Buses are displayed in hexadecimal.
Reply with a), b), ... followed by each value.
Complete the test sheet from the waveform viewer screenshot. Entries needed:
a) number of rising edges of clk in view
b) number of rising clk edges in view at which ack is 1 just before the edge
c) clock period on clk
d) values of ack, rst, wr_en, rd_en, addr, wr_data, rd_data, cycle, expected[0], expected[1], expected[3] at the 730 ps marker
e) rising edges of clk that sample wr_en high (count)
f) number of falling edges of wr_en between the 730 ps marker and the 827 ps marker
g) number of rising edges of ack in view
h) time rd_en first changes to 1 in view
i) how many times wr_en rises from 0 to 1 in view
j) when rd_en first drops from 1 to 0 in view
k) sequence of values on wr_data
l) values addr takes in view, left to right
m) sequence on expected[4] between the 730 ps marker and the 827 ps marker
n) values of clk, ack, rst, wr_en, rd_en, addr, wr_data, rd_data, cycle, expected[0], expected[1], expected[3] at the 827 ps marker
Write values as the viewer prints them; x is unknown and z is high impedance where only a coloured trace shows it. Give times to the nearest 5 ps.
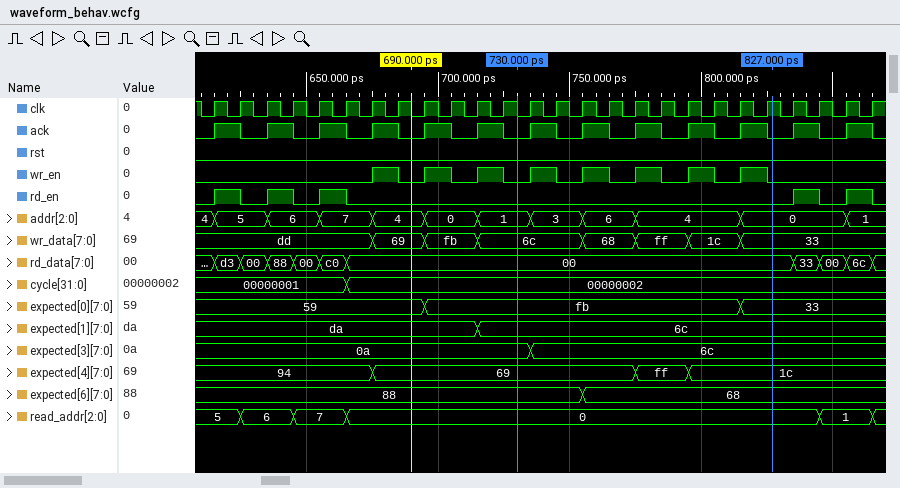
a) 26
b) 13
c) 10 ps
d) ack=0, rst=0, wr_en=0, rd_en=0, addr=1, wr_data=6c, rd_data=00, cycle=00000002, expected[0]=fb, expected[1]=6c, expected[3]=0a
e) 8
f) 5
g) 13
h) 615 ps
i) 8
j) 625 ps
k) dd, 69, fb, 6c, 68, ff, 1c, 33
l) 4, 5, 6, 7, 4, 0, 1, 3, 6, 4, 0, 1
m) 69, ff, 1c
n) clk=1, ack=0, rst=0, wr_en=0, rd_en=0, addr=0, wr_data=33, rd_data=00, cycle=00000002, expected[0]=33, expected[1]=6c, expected[3]=6c
